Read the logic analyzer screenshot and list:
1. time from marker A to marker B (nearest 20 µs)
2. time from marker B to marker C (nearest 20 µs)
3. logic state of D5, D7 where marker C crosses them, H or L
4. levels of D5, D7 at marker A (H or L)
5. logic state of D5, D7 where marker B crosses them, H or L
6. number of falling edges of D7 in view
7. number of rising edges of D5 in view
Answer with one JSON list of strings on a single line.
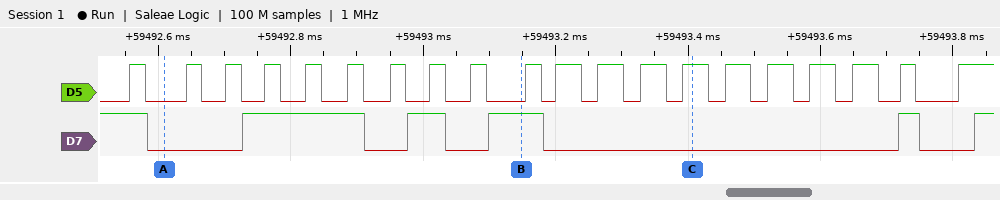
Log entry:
["540 µs", "260 µs", "D5=H, D7=L", "D5=L, D7=L", "D5=L, D7=H", "5", "20"]
